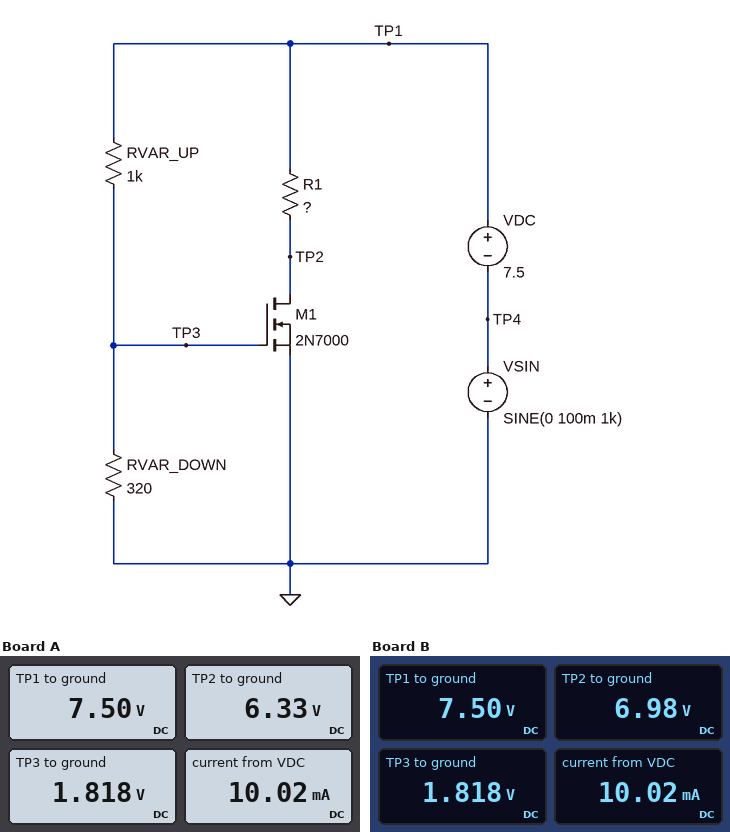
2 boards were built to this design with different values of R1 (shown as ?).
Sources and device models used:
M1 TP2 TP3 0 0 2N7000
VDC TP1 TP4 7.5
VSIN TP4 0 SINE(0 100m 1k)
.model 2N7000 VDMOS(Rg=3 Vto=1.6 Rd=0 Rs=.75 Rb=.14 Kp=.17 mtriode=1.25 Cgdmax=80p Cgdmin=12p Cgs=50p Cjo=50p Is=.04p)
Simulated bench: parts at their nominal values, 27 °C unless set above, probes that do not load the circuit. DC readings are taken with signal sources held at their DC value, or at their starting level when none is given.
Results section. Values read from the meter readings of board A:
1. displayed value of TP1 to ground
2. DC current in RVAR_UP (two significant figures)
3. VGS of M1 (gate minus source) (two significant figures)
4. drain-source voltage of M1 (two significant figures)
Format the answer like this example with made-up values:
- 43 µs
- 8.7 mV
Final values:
- 7.50 V
- 5.7 mA
- 1.8 V
- 6.3 V
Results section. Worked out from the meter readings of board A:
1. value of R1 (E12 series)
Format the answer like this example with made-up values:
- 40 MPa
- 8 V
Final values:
- 270 Ω
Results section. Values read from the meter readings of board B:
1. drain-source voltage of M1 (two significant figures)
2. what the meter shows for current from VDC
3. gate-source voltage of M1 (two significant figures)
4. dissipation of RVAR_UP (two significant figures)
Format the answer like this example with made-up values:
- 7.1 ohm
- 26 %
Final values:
- 7.0 V
- 10.02 mA
- 1.8 V
- 32 mW
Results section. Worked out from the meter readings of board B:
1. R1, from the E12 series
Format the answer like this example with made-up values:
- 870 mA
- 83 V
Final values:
- 120 Ω
